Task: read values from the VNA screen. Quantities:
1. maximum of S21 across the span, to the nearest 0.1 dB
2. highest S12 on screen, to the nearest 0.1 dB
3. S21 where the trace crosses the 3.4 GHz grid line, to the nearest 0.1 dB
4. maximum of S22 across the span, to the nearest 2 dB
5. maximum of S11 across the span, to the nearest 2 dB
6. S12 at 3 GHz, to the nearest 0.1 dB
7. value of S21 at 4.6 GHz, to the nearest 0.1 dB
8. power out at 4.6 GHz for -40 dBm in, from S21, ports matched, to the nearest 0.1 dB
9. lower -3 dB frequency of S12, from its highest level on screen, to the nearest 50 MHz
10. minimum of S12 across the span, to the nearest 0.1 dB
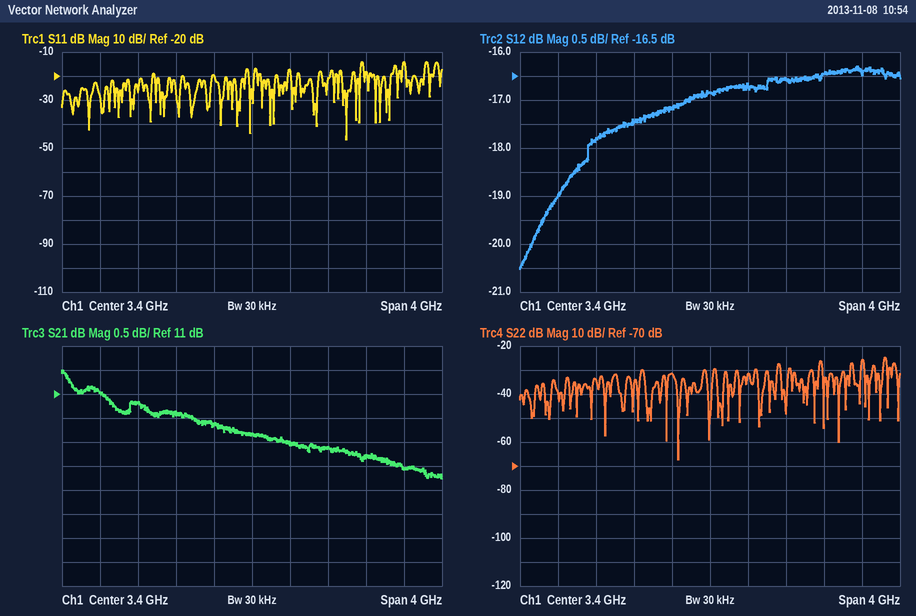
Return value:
11.5 dB
-16.3 dB
10.2 dB
-24 dB
-14 dB
-17.2 dB
9.7 dB
-30.3 dBm
1.70 GHz
-20.5 dB
